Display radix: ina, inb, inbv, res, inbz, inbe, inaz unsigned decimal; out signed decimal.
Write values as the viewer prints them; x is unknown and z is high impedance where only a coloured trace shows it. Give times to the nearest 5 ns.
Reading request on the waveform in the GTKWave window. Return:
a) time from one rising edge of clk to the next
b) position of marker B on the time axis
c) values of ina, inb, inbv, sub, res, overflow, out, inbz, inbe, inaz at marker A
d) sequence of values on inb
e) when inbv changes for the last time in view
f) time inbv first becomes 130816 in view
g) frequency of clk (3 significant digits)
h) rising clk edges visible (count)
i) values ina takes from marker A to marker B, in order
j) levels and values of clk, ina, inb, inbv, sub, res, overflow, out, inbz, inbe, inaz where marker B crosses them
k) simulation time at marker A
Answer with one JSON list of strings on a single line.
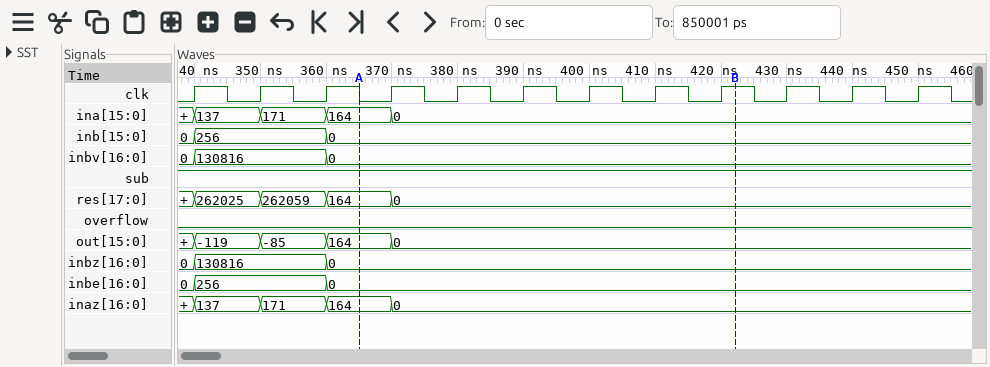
["10 ns", "420 ns", "ina=164, inb=0, inbv=0, sub=1, res=164, overflow=0, out=164, inbz=0, inbe=0, inaz=164", "0, 256, 0", "360 ns", "340 ns", "100 MHz", "12", "164, 0", "clk=1, ina=0, inb=0, inbv=0, sub=1, res=0, overflow=0, out=0, inbz=0, inbe=0, inaz=0", "365 ns"]
